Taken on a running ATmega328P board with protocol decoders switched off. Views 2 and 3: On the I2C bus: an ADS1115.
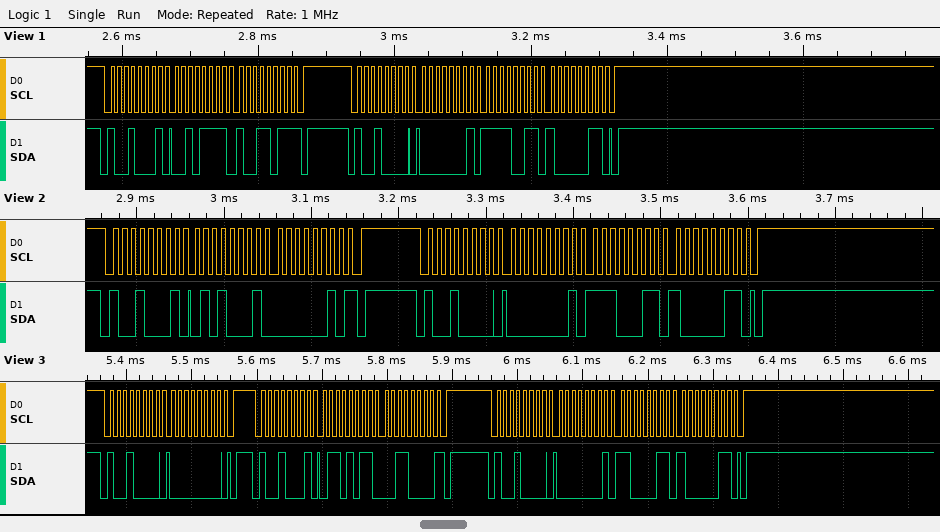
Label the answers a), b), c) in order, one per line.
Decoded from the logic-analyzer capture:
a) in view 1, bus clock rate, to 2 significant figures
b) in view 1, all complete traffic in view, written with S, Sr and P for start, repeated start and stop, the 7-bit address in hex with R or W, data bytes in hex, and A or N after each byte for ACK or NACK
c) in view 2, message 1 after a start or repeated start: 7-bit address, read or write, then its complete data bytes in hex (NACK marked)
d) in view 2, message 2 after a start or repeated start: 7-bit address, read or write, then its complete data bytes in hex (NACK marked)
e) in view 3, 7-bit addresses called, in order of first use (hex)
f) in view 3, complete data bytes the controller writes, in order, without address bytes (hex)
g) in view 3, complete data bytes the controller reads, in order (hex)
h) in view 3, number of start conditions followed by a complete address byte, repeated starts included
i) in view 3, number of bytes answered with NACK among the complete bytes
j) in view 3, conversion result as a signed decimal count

a) 100 kHz
b) S 48R A 2F A 9B N P S 48W A 01 A F3 A 83 A P
c) 0x48 read: 51 02 NACK
d) 0x48 write: 01 E3 83
e) 0x48
f) 00 01 C3 83
g) 6B 30
h) 3
i) 1
j) 27440
